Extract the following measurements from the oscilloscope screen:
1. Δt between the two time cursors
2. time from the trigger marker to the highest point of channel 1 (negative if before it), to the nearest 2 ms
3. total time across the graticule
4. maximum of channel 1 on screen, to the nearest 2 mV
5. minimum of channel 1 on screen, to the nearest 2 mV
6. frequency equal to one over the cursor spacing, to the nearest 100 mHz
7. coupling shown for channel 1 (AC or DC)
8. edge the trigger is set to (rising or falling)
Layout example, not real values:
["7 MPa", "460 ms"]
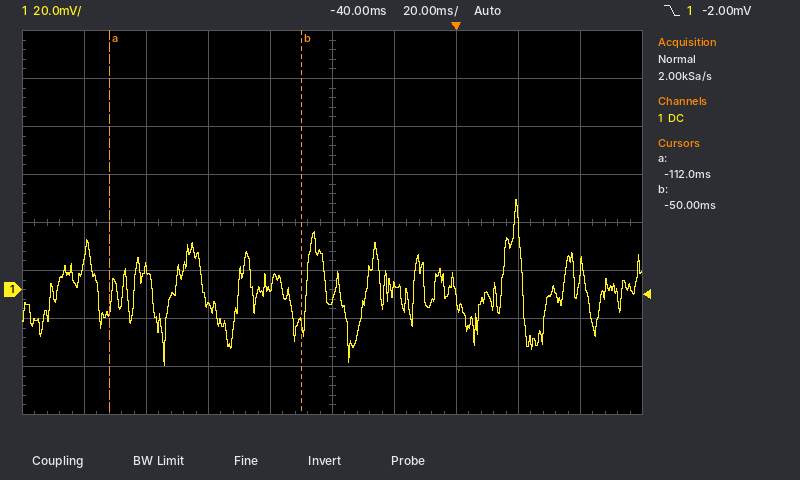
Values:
["62 ms", "+20 ms", "200 ms", "38 mV", "-32 mV", "16.1 Hz", "DC", "falling"]
